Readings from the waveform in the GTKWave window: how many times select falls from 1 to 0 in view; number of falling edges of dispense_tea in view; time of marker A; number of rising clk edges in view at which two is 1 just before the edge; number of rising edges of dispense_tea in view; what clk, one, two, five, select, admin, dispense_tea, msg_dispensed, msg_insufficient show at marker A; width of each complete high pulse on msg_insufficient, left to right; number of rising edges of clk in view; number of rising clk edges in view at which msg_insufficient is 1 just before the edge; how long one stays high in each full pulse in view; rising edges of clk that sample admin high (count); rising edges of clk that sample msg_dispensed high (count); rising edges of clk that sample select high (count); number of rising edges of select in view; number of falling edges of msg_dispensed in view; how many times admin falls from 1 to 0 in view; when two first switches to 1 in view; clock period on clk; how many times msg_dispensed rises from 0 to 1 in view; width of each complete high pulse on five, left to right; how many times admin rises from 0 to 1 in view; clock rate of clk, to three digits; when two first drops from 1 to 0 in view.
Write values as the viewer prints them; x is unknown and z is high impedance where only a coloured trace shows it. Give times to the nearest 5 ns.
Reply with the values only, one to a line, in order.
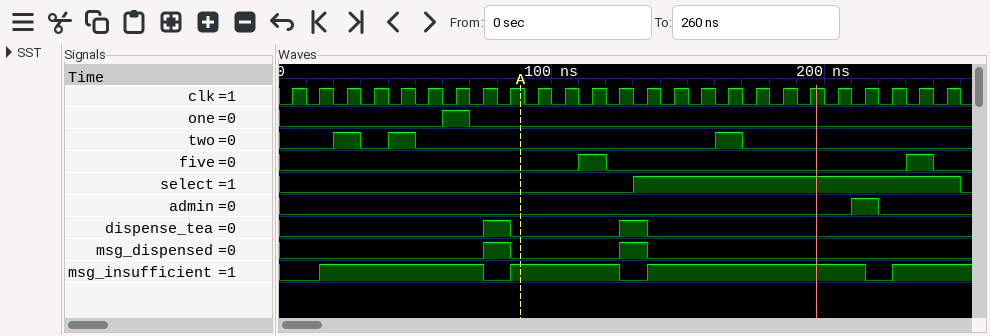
1
2
90 ns
3
2
clk=1, one=0, two=0, five=0, select=0, admin=0, dispense_tea=0, msg_dispensed=0, msg_insufficient=1
60 ns, 40 ns, 80 ns
25
20
10 ns
1
2
12
1
2
1
20 ns
10 ns
2
10 ns, 10 ns
1
100 MHz
30 ns
